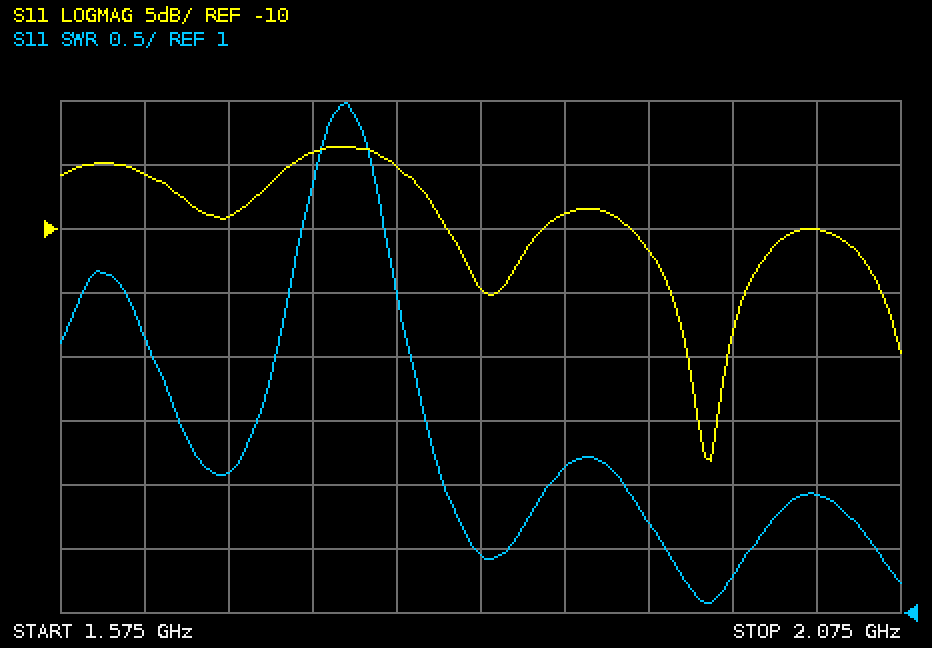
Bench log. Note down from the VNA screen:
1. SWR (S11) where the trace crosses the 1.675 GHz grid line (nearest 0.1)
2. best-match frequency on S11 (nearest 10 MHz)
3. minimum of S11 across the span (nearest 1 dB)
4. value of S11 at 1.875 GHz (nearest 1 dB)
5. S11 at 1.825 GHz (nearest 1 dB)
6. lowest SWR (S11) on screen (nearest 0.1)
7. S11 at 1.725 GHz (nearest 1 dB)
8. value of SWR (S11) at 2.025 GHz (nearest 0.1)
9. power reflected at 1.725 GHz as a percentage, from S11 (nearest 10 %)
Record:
2.1
1.96 GHz
-28 dB
-9 dB
-15 dB
1.1
-4 dB
1.9
40 %
